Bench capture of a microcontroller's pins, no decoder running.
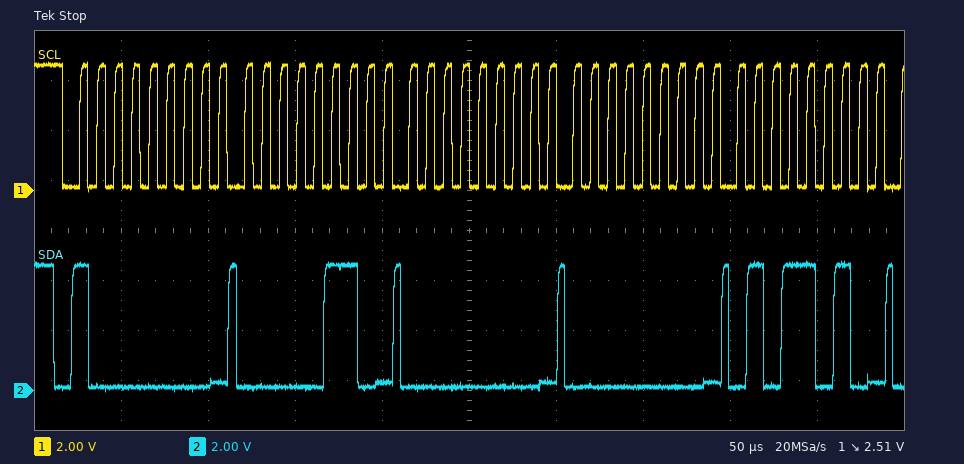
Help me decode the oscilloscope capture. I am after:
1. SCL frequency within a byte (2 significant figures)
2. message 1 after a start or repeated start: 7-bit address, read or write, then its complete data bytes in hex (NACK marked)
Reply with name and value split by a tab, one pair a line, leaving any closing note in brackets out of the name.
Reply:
SCL frequency within a byte	100 kHz
message 1 after a start or repeated start: 7-bit address, read or write, then its complete data bytes in hex	0x40 write: 06 00 00 5A
